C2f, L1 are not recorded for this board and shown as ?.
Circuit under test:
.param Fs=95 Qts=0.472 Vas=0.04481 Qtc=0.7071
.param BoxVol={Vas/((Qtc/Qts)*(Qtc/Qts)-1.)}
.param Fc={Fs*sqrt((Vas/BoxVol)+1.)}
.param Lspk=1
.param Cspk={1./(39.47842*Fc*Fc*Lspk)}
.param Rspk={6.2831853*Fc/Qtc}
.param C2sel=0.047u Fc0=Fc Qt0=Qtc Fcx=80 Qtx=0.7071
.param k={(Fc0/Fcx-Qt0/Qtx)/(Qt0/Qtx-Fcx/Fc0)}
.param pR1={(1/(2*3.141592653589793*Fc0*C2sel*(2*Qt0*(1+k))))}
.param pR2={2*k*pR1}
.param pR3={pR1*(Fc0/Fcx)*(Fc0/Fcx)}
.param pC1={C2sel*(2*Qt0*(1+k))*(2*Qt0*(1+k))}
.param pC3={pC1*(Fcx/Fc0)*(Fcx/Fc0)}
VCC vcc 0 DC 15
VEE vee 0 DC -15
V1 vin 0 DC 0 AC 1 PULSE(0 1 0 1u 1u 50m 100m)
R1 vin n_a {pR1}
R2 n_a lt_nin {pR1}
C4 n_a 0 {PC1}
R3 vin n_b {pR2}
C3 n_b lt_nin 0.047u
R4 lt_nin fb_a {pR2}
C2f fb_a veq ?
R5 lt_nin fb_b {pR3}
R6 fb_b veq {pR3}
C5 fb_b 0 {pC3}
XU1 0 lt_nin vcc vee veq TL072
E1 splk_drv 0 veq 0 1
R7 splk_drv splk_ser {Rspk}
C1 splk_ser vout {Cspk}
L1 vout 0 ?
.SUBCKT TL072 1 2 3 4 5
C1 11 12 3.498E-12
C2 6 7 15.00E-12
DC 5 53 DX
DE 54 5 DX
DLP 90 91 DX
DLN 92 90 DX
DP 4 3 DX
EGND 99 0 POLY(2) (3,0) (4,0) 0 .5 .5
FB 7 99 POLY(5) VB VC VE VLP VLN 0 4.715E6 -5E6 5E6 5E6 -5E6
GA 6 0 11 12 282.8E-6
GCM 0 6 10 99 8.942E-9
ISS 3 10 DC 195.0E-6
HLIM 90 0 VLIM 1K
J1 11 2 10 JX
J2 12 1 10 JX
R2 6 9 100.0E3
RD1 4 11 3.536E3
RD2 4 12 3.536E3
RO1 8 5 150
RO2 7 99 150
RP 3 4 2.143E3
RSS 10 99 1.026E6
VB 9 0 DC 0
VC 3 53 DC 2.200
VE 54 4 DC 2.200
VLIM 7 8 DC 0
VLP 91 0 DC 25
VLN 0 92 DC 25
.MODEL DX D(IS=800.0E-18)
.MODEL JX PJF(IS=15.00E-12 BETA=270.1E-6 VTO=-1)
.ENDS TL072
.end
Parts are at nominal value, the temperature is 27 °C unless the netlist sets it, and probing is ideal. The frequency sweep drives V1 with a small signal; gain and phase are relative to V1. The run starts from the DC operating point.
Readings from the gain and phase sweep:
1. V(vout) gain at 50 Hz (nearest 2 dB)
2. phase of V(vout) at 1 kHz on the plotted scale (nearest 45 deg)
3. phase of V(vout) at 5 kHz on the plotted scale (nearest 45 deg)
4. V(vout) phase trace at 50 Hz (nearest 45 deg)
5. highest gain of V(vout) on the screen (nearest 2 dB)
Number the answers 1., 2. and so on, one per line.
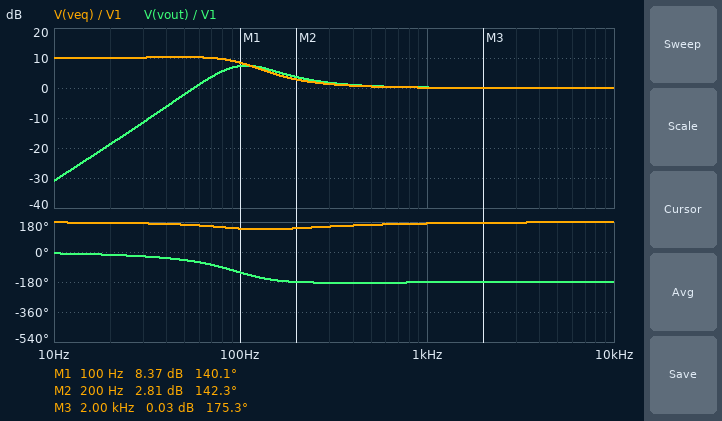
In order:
1. -2 dB
2. -180 deg
3. -180 deg
4. -45 deg
5. 8 dB
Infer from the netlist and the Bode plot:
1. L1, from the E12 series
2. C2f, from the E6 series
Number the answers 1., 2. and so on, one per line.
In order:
1. 1.8 H
2. 33 nF
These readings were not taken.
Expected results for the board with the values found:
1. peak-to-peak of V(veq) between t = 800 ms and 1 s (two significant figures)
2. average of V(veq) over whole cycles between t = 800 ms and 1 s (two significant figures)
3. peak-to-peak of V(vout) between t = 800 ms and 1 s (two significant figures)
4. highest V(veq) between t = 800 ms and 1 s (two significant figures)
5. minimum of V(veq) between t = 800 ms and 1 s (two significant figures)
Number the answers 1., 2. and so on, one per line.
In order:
1. 3.6 V
2. -1.6 V
3. 2.1 V
4. 230 mV
5. -3.4 V
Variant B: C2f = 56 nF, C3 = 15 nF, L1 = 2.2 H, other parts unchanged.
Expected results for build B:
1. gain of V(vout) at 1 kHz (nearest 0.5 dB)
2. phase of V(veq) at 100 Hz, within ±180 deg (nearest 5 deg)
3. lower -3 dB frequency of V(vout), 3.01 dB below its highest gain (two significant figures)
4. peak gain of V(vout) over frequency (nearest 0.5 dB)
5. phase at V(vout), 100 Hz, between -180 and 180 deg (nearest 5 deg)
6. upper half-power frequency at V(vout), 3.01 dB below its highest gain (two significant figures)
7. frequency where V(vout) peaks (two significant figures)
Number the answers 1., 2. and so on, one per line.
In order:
1. -1.0 dB
2. 115 deg
3. 62 Hz
4. 4.5 dB
5. -160 deg
6. 130 Hz
7. 91 Hz
